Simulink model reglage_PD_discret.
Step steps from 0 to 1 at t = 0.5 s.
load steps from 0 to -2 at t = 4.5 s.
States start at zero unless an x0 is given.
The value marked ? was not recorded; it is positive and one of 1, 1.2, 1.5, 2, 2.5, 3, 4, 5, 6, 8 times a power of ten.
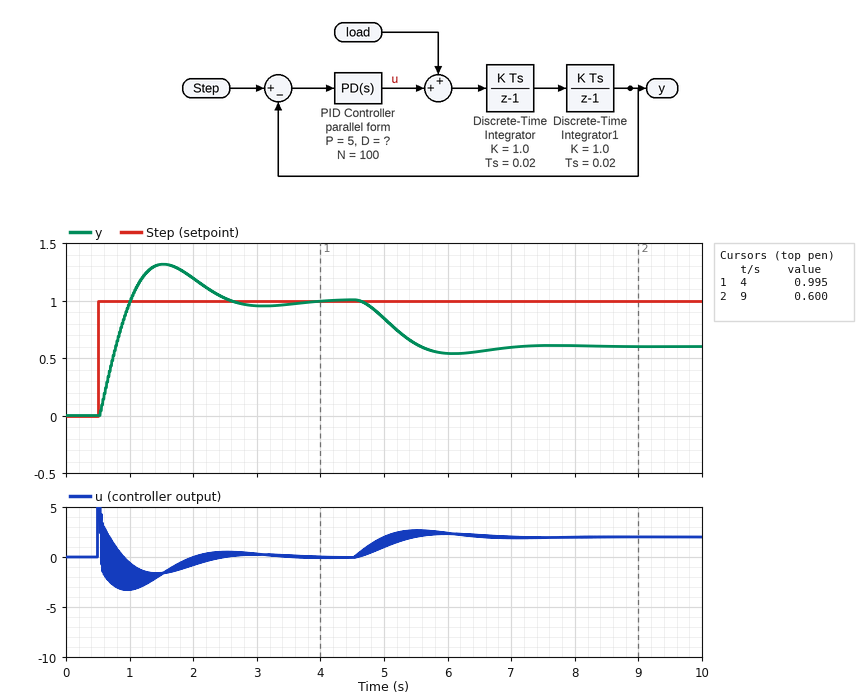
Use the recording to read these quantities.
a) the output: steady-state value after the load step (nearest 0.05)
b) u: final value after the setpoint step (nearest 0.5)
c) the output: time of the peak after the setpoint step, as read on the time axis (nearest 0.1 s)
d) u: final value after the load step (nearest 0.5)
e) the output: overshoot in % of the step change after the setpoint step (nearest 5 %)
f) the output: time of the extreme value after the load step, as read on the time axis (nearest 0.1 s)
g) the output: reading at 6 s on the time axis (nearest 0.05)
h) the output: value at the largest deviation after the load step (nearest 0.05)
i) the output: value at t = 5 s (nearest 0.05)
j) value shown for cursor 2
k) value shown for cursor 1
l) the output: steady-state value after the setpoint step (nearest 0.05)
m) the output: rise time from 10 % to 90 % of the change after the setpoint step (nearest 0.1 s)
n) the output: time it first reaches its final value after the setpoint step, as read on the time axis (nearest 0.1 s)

0.60
0.0
1.5 s
2.0
30 %
6.1 s
0.55
0.55
0.85
0.600
0.995
1.00
0.4 s
1.0 s
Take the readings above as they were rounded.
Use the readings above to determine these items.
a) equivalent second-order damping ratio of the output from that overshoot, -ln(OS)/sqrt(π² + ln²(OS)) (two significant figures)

0.36
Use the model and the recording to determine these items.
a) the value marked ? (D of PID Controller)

1
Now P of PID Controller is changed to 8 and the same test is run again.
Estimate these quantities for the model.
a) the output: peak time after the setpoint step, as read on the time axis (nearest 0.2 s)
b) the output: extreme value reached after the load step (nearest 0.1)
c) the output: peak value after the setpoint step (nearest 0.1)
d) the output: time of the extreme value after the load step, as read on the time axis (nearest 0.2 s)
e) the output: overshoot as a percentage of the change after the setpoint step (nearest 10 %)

1.4 s
0.7
1.4
5.6 s
40 %
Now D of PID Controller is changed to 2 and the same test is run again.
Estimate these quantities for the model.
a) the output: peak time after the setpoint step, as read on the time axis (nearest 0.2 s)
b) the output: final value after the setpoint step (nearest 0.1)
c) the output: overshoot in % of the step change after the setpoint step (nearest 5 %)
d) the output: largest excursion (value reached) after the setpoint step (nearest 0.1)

1.2 s
1.0
15 %
1.1
